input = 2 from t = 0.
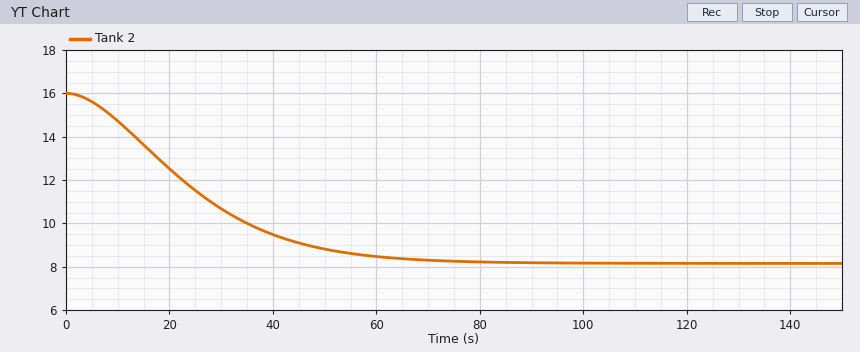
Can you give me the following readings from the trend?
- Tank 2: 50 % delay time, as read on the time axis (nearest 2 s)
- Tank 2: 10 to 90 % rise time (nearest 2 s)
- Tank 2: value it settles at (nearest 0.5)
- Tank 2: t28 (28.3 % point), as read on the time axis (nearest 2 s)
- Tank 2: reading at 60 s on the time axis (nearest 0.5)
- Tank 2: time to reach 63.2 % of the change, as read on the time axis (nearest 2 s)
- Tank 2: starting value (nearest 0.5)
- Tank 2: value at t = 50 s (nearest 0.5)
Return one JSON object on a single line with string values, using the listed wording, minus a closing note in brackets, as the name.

{"Tank 2: 50 % delay time, as read on the time axis": "22 s", "Tank 2: 10 to 90 % rise time": "40 s", "Tank 2: value it settles at": "8.0", "Tank 2: t28 (28.3 % point), as read on the time axis": "14 s", "Tank 2: reading at 60 s on the time axis": "8.5", "Tank 2: time to reach 63.2 % of the change, as read on the time axis": "28 s", "Tank 2: starting value": "16.0", "Tank 2: value at t = 50 s": "9.0"}
